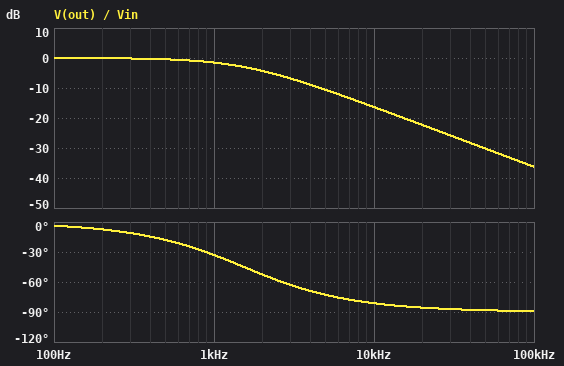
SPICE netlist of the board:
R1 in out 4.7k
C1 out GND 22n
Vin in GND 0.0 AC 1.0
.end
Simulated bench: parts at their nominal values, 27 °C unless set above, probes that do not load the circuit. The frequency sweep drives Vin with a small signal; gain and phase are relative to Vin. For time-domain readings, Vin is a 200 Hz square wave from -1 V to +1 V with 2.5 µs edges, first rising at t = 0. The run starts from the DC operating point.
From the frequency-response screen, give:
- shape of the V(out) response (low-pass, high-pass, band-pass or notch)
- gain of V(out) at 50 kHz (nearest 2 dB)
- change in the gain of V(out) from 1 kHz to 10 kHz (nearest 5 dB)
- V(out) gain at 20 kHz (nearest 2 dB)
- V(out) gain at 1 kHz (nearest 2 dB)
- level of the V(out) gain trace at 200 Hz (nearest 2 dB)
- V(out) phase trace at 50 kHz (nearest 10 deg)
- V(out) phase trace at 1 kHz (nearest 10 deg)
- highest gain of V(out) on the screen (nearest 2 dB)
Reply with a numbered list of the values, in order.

1. low-pass
2. -30 dB
3. -15 dB
4. -22 dB
5. -2 dB
6. 0 dB
7. -90 deg
8. -30 deg
9. 0 dB
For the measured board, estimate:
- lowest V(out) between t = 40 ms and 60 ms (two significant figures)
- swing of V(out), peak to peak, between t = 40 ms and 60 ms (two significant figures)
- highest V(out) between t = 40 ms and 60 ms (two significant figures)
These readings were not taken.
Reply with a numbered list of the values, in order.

1. -1.0 V
2. 2.0 V
3. 1.0 V
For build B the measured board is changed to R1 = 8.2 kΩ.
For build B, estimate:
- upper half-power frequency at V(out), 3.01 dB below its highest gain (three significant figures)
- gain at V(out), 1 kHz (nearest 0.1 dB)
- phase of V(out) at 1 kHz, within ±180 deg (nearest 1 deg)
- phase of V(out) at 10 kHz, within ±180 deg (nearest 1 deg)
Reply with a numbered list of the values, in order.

1. 882 Hz
2. -3.6 dB
3. -49 deg
4. -85 deg
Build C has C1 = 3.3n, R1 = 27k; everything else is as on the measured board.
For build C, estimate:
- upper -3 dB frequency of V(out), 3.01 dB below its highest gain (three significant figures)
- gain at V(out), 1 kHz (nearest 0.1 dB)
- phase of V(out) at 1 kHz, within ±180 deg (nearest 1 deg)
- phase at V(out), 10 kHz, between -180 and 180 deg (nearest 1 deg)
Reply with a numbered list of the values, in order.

1. 1.79 kHz
2. -1.2 dB
3. -29 deg
4. -80 deg
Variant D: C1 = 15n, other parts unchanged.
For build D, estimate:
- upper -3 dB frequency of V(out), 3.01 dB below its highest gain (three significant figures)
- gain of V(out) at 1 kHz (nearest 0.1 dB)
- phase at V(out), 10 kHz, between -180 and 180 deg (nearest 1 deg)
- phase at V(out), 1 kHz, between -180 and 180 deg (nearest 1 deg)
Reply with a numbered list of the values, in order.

1. 2.26 kHz
2. -0.8 dB
3. -77 deg
4. -24 deg
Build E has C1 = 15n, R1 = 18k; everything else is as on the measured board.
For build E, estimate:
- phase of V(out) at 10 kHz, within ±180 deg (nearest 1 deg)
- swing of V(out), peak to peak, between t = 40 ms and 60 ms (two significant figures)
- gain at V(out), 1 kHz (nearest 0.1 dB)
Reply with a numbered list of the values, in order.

1. -87 deg
2. 2.0 V
3. -5.9 dB
